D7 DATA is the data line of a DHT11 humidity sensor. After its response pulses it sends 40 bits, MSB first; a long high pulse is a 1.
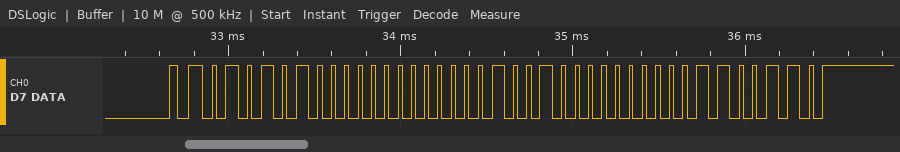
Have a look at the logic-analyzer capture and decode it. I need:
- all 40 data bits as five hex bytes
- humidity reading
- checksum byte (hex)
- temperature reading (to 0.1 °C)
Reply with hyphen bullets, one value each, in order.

- 54 00 12 00 66
- 84 %
- 0x66
- 18.0 °C
